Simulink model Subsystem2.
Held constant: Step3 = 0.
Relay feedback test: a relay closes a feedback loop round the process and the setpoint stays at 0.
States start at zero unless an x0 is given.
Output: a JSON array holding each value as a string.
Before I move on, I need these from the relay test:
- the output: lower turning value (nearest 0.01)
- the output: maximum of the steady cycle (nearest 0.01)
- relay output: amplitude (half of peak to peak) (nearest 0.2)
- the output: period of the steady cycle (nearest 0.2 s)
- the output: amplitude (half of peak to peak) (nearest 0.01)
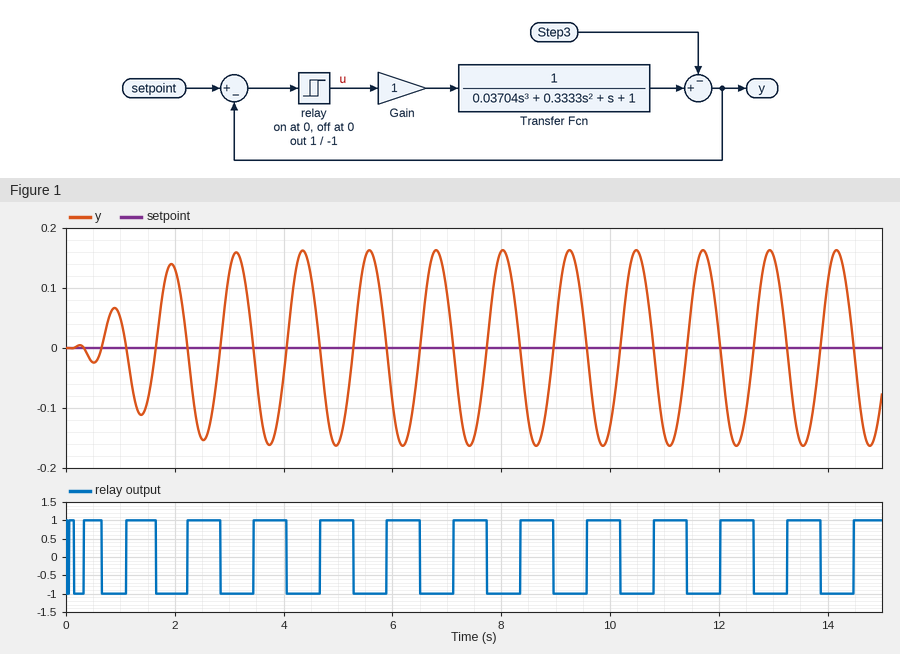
["-0.16", "0.16", "1.0", "1.2 s", "0.16"]
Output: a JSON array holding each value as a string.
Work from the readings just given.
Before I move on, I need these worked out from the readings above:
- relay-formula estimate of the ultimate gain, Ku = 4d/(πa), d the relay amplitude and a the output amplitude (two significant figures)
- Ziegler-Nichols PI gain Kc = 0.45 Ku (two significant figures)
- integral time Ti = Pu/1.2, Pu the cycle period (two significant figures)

["8.0", "3.6", "1.0 s"]
